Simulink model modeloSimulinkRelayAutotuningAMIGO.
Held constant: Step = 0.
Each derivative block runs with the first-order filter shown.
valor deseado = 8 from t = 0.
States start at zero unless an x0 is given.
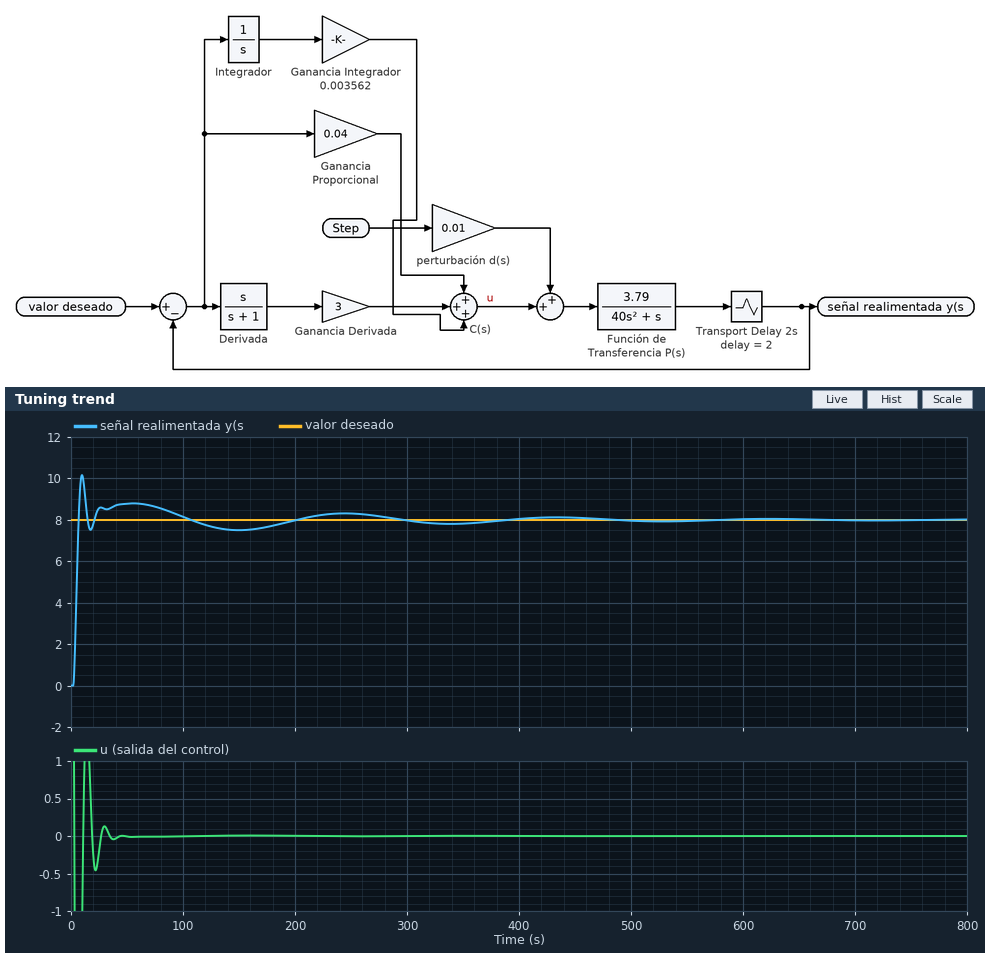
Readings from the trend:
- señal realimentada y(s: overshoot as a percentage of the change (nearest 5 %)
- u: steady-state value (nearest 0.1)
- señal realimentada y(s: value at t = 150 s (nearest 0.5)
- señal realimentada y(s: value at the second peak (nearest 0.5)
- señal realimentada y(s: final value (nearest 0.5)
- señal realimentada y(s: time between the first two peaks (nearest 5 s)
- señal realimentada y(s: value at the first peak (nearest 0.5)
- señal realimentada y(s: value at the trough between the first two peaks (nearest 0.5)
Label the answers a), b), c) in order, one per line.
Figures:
a) 25 %
b) 0.0
c) 7.5
d) 9.0
e) 8.0
f) 45 s
g) 10.0
h) 7.5
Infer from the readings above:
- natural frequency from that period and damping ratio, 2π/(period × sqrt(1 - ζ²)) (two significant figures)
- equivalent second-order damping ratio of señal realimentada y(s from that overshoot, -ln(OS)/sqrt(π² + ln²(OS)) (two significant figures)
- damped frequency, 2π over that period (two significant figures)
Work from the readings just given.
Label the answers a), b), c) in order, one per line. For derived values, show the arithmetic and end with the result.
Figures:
a) 2π / (45 × sqrt(1 - 0.4²)) = 0.15 rad/s
b) ln(0.25) = -1.386; 1.386 / sqrt(9.870 + 1.922) = 0.40
c) 2π / 45 = 0.14 rad/s
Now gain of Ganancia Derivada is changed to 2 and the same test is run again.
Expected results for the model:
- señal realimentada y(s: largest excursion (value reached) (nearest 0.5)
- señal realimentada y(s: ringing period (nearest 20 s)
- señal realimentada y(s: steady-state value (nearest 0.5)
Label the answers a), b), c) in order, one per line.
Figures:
a) 9.5
b) 160 s
c) 8.0
